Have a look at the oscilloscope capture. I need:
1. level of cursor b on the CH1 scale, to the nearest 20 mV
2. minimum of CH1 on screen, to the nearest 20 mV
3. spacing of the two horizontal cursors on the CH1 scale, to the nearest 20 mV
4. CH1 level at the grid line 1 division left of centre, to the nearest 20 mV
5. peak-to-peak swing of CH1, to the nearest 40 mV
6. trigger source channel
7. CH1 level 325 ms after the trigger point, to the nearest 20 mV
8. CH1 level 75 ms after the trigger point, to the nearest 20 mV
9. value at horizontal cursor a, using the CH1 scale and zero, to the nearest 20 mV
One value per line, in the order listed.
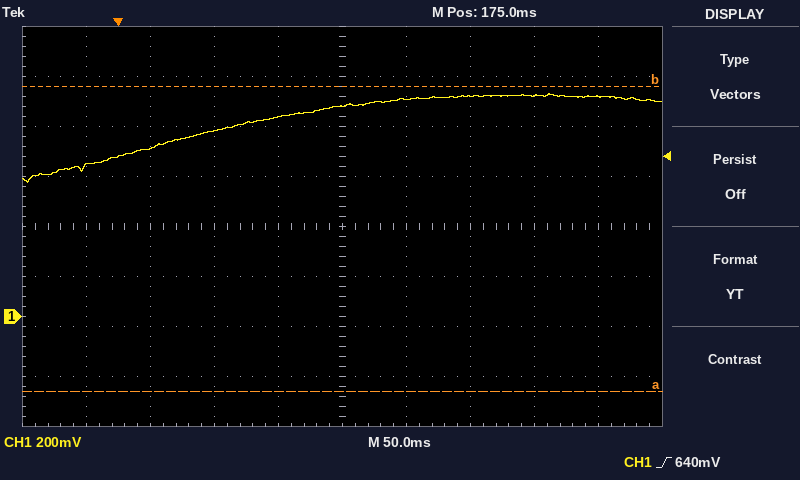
920 mV
540 mV
1.22 V
800 mV
360 mV
CH1
880 mV
740 mV
-300 mV
